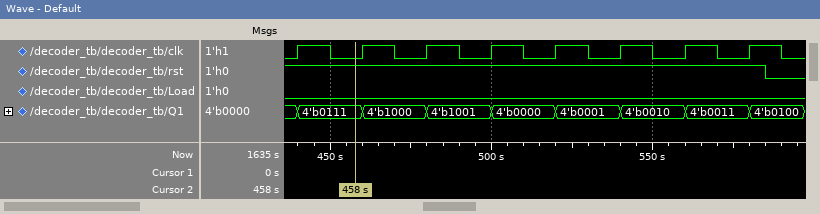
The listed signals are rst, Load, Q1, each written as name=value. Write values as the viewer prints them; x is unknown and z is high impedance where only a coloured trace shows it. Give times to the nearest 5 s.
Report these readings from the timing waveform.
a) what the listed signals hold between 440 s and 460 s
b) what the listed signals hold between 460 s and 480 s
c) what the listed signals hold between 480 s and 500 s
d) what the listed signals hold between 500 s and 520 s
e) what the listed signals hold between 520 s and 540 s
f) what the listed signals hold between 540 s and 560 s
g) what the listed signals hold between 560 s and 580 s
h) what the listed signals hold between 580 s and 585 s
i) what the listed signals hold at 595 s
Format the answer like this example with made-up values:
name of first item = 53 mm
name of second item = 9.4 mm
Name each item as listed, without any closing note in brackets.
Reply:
what the listed signals hold between 440 s and 460 s = rst=1, Load=0, Q1=4'b0111
what the listed signals hold between 460 s and 480 s = rst=1, Load=0, Q1=4'b1000
what the listed signals hold between 480 s and 500 s = rst=1, Load=0, Q1=4'b1001
what the listed signals hold between 500 s and 520 s = rst=1, Load=0, Q1=4'b0000
what the listed signals hold between 520 s and 540 s = rst=1, Load=0, Q1=4'b0001
what the listed signals hold between 540 s and 560 s = rst=1, Load=0, Q1=4'b0010
what the listed signals hold between 560 s and 580 s = rst=1, Load=0, Q1=4'b0011
what the listed signals hold between 580 s and 585 s = rst=1, Load=0, Q1=4'b0100
what the listed signals hold at 595 s = rst=0, Load=0, Q1=4'b0100
